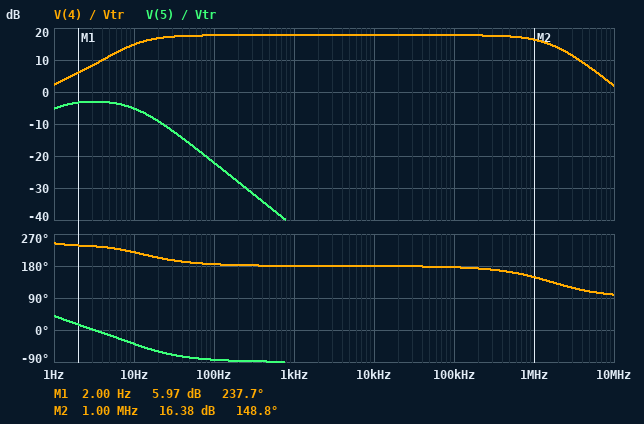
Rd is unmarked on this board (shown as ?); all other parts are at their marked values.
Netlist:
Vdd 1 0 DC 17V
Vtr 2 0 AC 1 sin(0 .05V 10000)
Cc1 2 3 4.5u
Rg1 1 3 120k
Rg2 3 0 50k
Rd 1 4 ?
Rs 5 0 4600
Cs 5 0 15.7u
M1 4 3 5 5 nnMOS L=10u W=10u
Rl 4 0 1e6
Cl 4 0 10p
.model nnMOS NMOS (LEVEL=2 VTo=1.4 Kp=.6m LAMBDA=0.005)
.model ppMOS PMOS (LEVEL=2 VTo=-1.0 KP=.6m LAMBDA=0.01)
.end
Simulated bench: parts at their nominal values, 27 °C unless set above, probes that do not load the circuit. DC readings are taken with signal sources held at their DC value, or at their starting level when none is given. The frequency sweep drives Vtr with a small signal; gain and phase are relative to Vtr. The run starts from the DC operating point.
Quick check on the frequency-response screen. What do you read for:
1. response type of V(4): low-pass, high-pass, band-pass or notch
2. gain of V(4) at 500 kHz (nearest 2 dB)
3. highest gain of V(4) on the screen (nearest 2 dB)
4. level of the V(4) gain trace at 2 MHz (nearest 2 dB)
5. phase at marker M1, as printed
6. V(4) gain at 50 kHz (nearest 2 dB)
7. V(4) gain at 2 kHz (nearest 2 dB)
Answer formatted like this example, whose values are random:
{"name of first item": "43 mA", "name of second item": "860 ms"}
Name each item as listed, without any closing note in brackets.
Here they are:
{"response type of V(4): low-pass, high-pass, band-pass or notch": "band-pass", "gain of V(4) at 500 kHz": "18 dB", "highest gain of V(4) on the screen": "18 dB", "level of the V(4) gain trace at 2 MHz": "14 dB", "phase at marker M1, as printed": "237.7 deg", "V(4) gain at 50 kHz": "18 dB", "V(4) gain at 2 kHz": "18 dB"}
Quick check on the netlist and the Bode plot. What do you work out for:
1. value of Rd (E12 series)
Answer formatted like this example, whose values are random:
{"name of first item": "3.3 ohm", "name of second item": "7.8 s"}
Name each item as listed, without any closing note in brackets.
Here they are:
{"value of Rd": "10 kΩ"}
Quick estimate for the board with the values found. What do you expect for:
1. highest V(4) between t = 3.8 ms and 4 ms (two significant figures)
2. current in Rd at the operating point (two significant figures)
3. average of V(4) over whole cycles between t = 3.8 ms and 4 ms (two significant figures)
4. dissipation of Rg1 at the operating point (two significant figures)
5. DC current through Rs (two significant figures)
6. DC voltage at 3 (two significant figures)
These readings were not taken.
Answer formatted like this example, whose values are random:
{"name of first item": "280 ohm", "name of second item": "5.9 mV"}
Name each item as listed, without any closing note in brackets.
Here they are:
{"highest V(4) between t = 3.8 ms and 4 ms": "12 V", "current in Rd at the operating point": "520 µA", "average of V(4) over whole cycles between t = 3.8 ms and 4 ms": "12 V", "dissipation of Rg1 at the operating point": "1.2 mW", "DC current through Rs": "510 µA", "DC voltage at 3": "5.0 V"}
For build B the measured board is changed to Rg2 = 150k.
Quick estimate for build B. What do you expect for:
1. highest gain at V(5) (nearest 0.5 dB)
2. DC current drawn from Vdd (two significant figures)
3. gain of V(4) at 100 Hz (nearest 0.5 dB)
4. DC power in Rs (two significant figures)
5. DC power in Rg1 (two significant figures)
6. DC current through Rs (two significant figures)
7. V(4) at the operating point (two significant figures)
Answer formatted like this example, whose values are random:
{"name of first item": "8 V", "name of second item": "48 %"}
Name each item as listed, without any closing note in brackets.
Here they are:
{"highest gain at V(5)": "-22.5 dB", "DC current drawn from Vdd": "1.2 mA", "gain of V(4) at 100 Hz": "-10.5 dB", "DC power in Rs": "5.7 mW", "DC power in Rg1": "480 µW", "DC current through Rs": "1.1 mA", "V(4) at the operating point": "5.8 V"}
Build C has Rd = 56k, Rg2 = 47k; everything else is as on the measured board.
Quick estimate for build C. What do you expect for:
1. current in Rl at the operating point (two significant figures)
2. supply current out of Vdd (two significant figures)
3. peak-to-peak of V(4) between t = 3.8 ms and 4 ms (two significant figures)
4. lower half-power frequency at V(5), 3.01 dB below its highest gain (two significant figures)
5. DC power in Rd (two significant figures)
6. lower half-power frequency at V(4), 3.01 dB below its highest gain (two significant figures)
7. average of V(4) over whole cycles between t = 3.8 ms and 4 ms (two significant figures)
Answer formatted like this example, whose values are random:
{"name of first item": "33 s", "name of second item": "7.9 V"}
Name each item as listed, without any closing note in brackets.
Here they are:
{"current in Rl at the operating point": "1.5 µA", "supply current out of Vdd": "380 µA", "peak-to-peak of V(4) between t = 3.8 ms and 4 ms": "12 mV", "lower half-power frequency at V(5), 3.01 dB below its highest gain": "620 mHz", "DC power in Rd": "4.3 mW", "lower half-power frequency at V(4), 3.01 dB below its highest gain": "1.2 Hz", "average of V(4) over whole cycles between t = 3.8 ms and 4 ms": "1.5 V"}
